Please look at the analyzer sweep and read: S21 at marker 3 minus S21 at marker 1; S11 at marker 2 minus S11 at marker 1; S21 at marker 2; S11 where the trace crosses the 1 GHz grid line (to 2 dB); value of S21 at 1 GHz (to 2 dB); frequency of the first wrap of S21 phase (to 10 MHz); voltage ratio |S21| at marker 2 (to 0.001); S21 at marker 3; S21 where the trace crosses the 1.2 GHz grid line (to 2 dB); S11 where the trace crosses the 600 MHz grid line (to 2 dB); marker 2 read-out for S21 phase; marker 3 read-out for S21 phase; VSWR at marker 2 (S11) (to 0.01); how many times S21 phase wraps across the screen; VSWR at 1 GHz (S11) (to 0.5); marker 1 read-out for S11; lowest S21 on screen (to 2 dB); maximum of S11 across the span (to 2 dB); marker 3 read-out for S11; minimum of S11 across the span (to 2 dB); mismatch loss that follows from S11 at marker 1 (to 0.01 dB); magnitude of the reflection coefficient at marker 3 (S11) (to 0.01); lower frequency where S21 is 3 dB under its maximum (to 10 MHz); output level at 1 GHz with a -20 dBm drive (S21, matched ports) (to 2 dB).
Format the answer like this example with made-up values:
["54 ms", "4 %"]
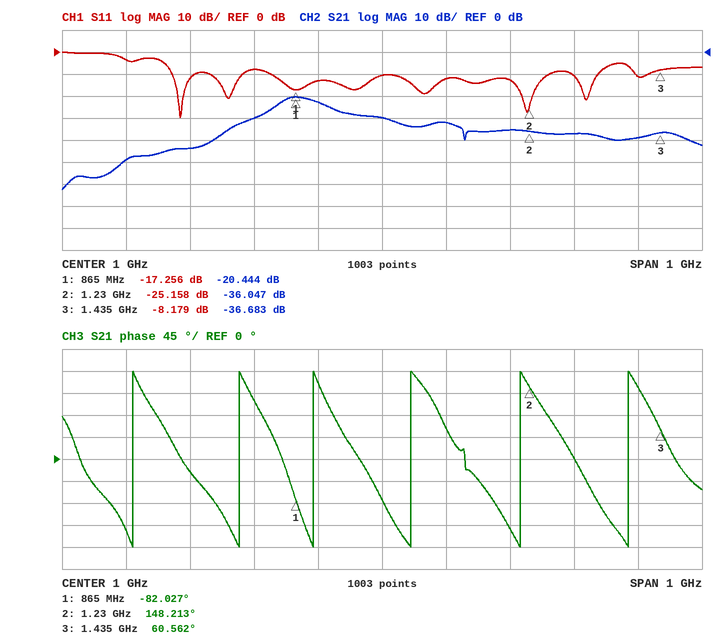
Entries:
["-16.239 dB", "-7.902 dB", "-36.047 dB", "-10 dB", "-30 dB", "610 MHz", "0.016", "-36.683 dB", "-36 dB", "-4 dB", "148.213°", "60.562°", "1.12", "6", "2.0", "-17.256 dB", "-62 dB", "0 dB", "-8.179 dB", "-30 dB", "0.08 dB", "0.39", "840 MHz", "-50 dBm"]
